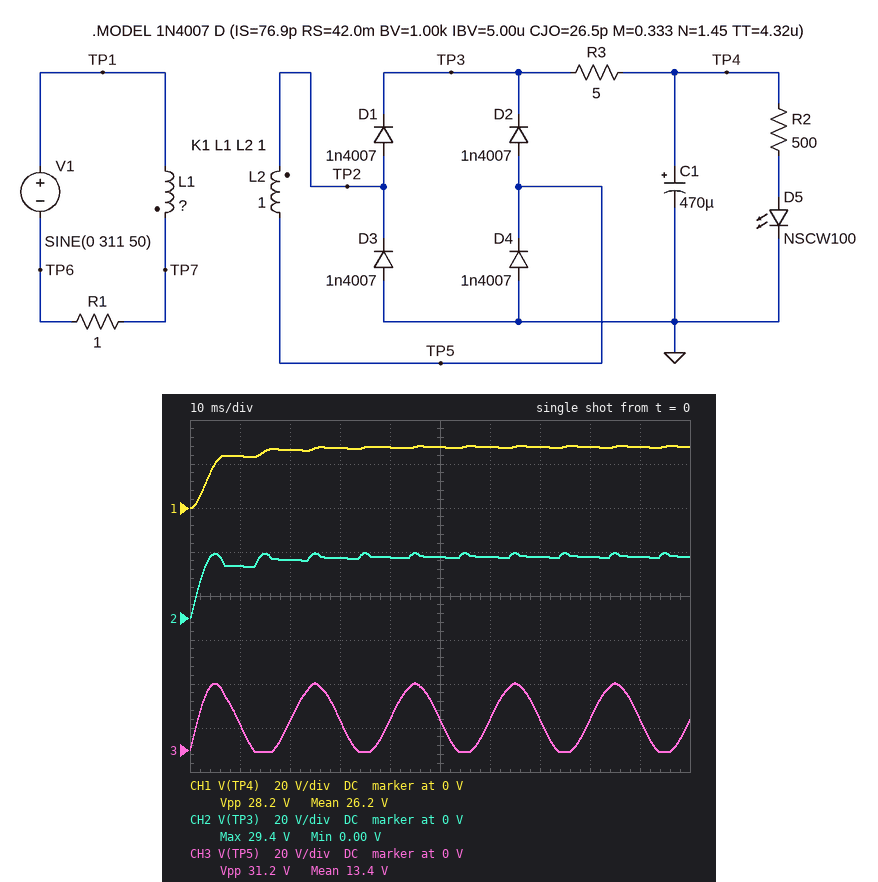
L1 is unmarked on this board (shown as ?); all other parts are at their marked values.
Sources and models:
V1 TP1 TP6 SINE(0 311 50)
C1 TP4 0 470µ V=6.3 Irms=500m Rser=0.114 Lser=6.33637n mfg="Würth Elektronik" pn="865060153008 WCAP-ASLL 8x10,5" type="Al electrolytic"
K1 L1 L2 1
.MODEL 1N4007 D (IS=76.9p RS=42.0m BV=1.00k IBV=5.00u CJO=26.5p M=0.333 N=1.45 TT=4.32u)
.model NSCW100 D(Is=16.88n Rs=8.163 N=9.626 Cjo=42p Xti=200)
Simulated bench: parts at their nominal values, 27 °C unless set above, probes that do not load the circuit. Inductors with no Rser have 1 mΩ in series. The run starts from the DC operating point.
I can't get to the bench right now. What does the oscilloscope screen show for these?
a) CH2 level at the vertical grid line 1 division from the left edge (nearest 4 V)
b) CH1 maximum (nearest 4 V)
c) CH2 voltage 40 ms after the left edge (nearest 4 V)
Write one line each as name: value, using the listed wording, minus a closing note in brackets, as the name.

CH2 level at the vertical grid line 1 division from the left edge: 24 V
CH1 maximum: 28 V
CH2 voltage 40 ms after the left edge: 28 V
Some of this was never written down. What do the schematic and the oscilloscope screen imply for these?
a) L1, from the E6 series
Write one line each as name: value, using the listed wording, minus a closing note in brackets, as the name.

L1, from the E6 series: 100 H
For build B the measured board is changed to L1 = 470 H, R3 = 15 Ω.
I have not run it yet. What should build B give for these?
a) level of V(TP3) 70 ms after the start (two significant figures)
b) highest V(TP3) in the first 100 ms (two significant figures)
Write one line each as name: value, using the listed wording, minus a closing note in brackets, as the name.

level of V(TP3) 70 ms after the start: 11 V
highest V(TP3) in the first 100 ms: 13 V
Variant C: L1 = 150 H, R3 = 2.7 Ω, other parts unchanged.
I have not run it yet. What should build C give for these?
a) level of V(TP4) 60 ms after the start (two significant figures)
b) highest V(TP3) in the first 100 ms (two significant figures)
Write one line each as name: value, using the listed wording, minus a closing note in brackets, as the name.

level of V(TP4) 60 ms after the start: 23 V
highest V(TP3) in the first 100 ms: 24 V
